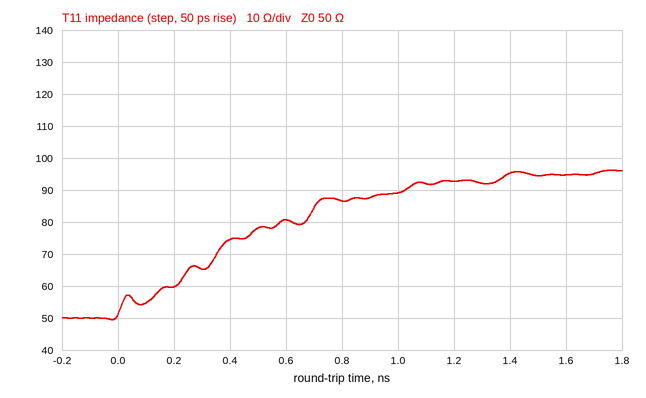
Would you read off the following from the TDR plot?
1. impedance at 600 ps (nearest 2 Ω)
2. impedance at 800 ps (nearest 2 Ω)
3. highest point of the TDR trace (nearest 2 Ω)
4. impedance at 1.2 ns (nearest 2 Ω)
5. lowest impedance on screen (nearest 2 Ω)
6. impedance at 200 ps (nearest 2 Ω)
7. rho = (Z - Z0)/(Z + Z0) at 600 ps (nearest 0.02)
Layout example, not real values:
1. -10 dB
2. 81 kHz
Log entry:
1. 80 Ω
2. 86 Ω
3. 96 Ω
4. 92 Ω
5. 50 Ω
6. 60 Ω
7. +0.24
